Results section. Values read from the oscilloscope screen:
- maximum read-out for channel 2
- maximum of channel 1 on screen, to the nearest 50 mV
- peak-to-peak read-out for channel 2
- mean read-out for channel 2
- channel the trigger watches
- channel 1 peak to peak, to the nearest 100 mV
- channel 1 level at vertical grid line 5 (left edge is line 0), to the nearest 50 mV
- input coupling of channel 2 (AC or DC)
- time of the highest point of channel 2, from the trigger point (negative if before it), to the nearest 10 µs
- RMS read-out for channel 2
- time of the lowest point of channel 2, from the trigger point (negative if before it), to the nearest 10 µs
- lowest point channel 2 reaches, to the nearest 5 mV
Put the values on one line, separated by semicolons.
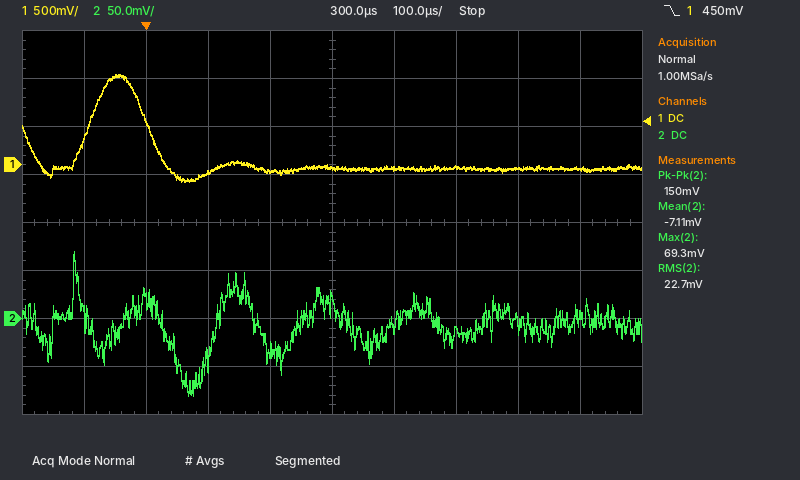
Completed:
69.3 mV; 950 mV; 150 mV; -7.11 mV; channel 1; 1.10 V; -50 mV; DC; -120 µs; 22.7 mV; +70 µs; -80 mV
